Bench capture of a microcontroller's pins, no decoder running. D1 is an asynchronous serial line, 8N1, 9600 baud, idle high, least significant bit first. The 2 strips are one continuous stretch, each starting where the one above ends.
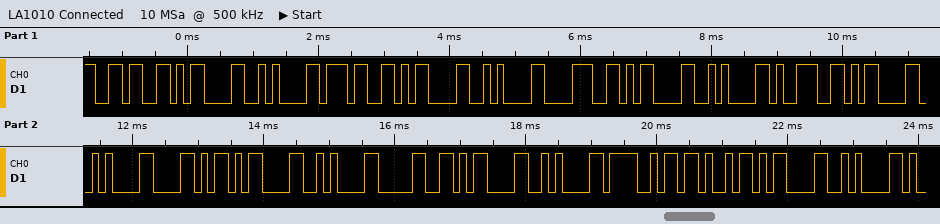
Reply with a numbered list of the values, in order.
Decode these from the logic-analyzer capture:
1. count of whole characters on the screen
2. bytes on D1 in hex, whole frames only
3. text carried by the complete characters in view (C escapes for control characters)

1. 22
2. 36 0D 0A 37 0D 0A 38 0D 0A 39 0D 0A 58 0D 0A 30 0D 0A 4F 4B 0D 0A
3. "6\r\n7\r\n8\r\n9\r\nX\r\n0\r\nOK\r\n"
